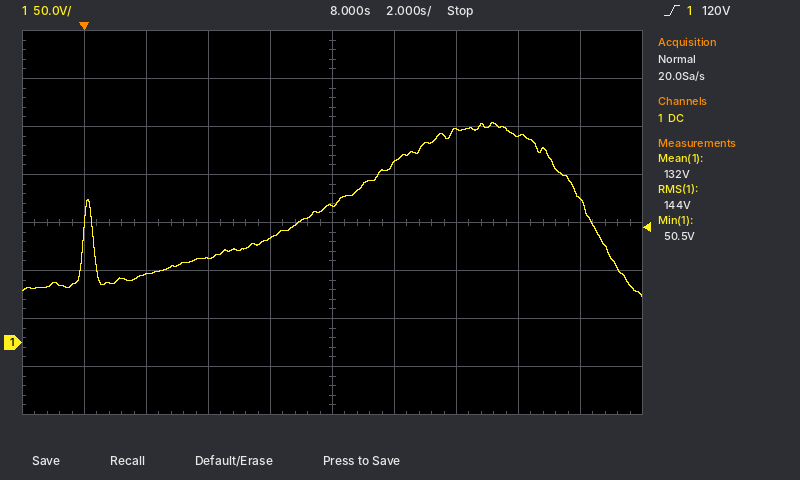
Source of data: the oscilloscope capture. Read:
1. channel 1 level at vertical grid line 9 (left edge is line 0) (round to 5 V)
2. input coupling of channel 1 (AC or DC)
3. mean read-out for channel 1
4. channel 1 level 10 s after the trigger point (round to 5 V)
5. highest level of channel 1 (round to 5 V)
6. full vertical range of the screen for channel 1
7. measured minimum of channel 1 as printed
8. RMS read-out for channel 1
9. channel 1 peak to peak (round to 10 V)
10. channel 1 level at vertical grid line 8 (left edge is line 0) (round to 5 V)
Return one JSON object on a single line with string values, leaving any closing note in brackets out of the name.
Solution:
{"channel 1 level at vertical grid line 9 (left edge is line 0)": "150 V", "input coupling of channel 1": "DC", "mean read-out for channel 1": "132 V", "channel 1 level 10 s after the trigger point": "185 V", "highest level of channel 1": "230 V", "full vertical range of the screen for channel 1": "400 V", "measured minimum of channel 1 as printed": "50.5 V", "RMS read-out for channel 1": "144 V", "channel 1 peak to peak": "180 V", "channel 1 level at vertical grid line 8 (left edge is line 0)": "215 V"}
